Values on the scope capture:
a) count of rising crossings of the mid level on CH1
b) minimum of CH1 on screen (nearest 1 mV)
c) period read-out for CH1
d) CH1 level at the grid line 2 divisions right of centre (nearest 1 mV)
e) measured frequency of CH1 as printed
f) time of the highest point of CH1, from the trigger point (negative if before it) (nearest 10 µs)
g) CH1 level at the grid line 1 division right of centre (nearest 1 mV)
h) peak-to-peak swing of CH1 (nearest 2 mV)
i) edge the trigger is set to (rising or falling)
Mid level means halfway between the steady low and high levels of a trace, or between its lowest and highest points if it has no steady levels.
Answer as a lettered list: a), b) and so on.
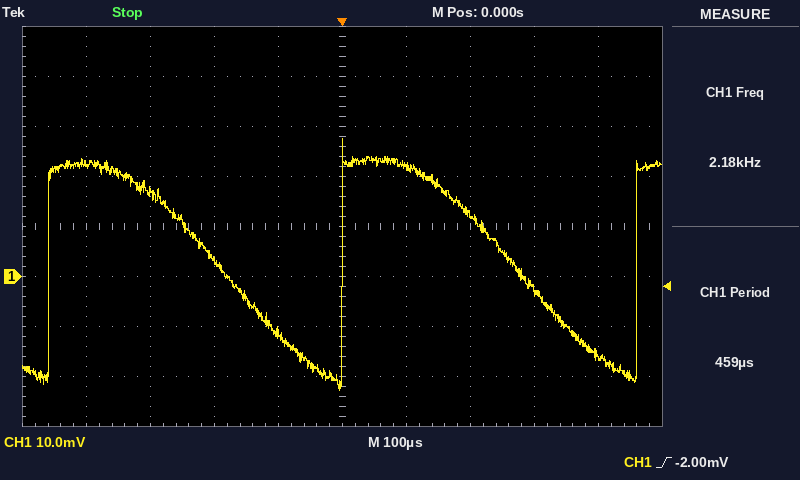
a) 3
b) -23 mV
c) 459 µs
d) 12 mV
e) 2.18 kHz
f) 0 µs
g) 22 mV
h) 50 mV
i) rising
